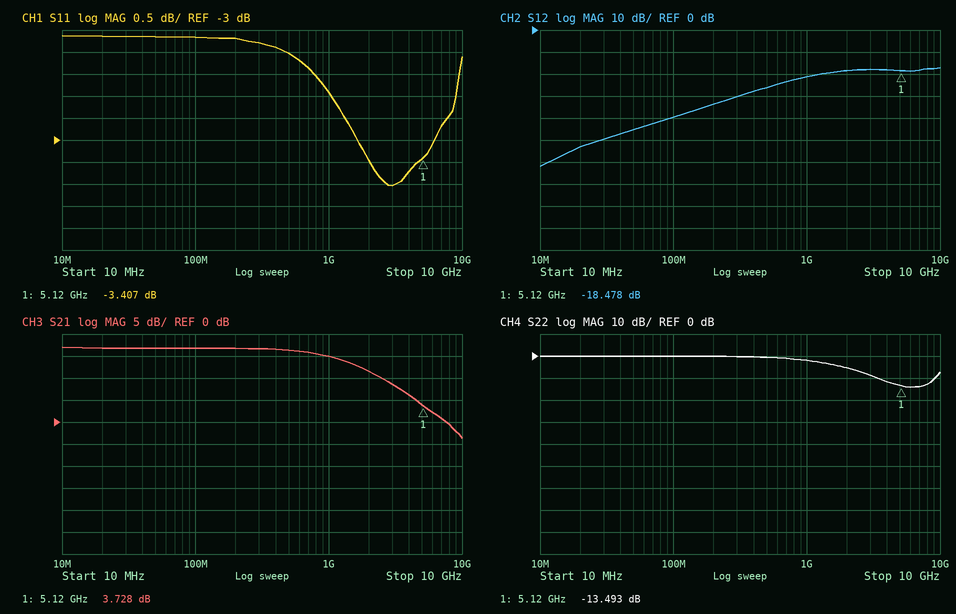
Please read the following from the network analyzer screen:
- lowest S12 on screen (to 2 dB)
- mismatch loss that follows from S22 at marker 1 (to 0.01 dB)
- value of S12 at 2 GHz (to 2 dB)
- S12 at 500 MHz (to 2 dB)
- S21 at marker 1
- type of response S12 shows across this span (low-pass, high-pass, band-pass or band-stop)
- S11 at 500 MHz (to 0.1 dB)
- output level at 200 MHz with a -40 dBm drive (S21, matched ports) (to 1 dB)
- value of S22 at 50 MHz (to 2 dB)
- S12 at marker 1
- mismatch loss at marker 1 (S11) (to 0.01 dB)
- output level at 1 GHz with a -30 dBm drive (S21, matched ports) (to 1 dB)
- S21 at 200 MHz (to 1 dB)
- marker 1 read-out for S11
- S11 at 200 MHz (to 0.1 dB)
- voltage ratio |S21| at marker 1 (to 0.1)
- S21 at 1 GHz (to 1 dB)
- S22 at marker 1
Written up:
-62 dB
0.20 dB
-18 dB
-26 dB
3.728 dB
high-pass
-1.0 dB
-23 dBm
0 dB
-18.478 dB
2.65 dB
-15 dBm
17 dB
-3.407 dB
-0.7 dB
1.5
15 dB
-13.493 dB
